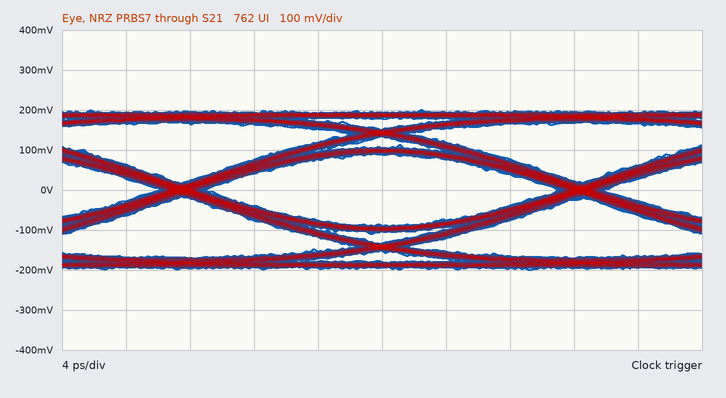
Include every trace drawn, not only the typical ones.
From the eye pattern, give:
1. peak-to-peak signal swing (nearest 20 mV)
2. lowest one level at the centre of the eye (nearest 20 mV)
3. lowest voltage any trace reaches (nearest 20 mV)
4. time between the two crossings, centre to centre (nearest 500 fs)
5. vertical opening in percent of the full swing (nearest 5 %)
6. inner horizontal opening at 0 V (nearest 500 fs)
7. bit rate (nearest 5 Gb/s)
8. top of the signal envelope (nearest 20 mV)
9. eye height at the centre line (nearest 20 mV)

400 mV
80 mV
-200 mV
25.0 ps
45 %
22.0 ps
40 Gb/s
200 mV
180 mV
